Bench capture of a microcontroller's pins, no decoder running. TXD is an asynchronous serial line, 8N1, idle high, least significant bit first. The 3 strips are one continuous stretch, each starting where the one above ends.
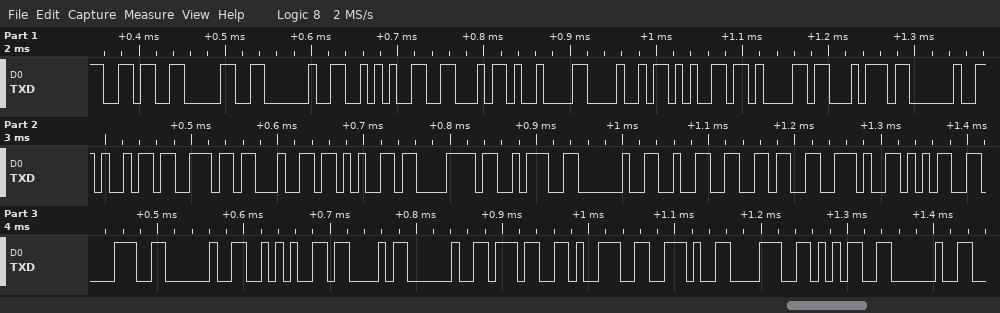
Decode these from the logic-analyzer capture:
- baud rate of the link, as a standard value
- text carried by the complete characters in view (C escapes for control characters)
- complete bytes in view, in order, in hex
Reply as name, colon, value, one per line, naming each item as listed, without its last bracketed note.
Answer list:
baud rate of the link, as a standard value: 115200 baud
text carried by the complete characters in view: "60 *F\tHeat index: 26.58 *C 79.85 "
complete bytes in view, in order, in hex: 36 30 20 2A 46 09 48 65 61 74 20 69 6E 64 65 78 3A 20 32 36 2E 35 38 20 2A 43 20 37 39 2E 38 35 20
